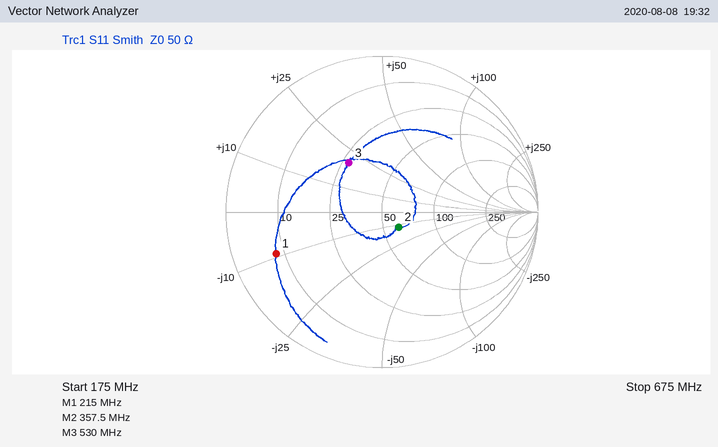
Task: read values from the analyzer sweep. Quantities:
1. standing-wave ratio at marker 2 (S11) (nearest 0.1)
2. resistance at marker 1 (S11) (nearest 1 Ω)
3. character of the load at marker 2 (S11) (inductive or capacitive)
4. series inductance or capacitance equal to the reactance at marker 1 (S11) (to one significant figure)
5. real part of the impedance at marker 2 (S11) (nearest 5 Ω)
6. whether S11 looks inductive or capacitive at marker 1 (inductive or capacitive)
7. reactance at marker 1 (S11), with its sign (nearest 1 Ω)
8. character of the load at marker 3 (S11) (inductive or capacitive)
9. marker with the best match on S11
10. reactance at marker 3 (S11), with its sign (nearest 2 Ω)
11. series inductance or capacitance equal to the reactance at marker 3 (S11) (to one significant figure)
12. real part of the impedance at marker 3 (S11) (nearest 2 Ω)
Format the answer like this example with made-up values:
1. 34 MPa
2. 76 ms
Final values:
1. 1.3
2. 8 Ω
3. capacitive
4. 80 pF
5. 60 Ω
6. capacitive
7. -9 Ω
8. inductive
9. marker 2
10. +20 Ω
11. 6 nH
12. 28 Ω
